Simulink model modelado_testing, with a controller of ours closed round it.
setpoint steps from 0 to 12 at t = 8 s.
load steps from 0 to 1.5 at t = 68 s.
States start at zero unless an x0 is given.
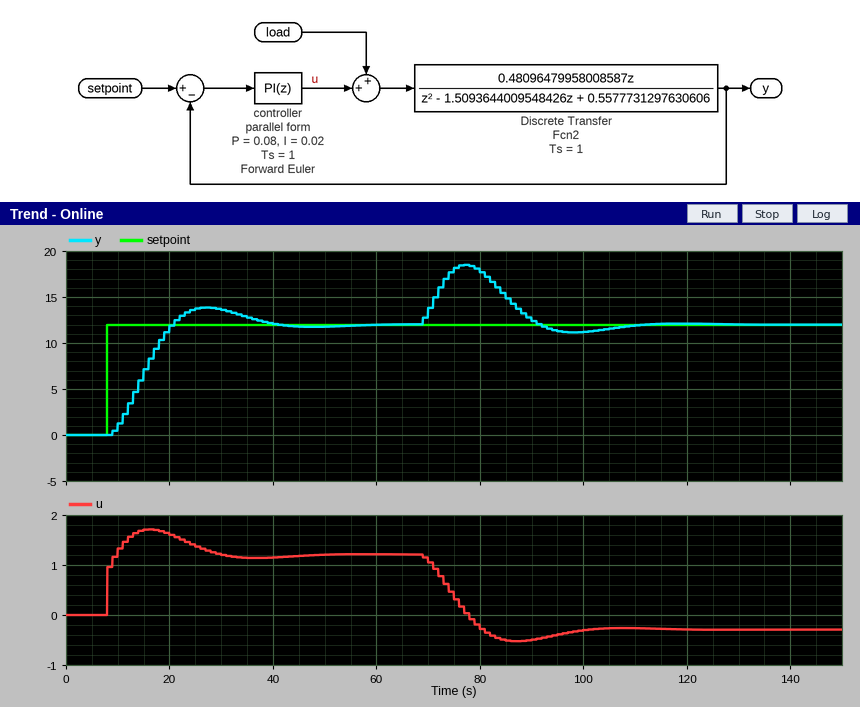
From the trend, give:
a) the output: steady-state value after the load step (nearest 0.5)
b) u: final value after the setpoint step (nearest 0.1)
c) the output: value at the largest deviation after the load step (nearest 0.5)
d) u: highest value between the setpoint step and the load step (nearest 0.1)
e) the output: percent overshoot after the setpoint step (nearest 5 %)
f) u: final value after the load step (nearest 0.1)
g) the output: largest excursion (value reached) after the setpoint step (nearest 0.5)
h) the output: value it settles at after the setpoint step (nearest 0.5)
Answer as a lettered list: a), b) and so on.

a) 12.0
b) 1.2
c) 18.5
d) 1.7
e) 15 %
f) -0.3
g) 14.0
h) 12.0
